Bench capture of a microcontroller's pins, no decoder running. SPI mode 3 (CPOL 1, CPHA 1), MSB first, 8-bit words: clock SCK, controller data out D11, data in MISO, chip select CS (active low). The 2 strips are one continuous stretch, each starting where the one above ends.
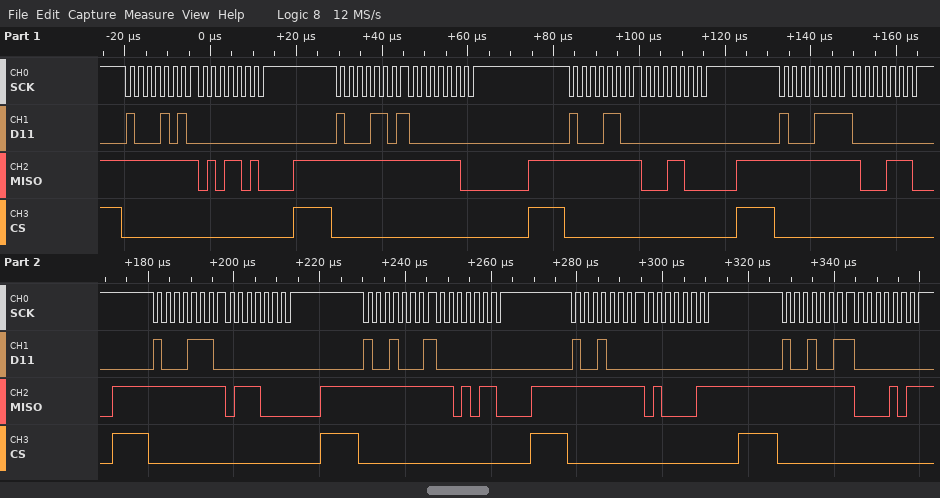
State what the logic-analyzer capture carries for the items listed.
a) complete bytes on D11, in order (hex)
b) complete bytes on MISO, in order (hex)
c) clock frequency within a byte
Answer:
8A 00 8D 00 8C 00 8F 00 8E 00 91 00 90 00 93 00
FF 5A FF FC FF 18 FF 8E FF 70 FF D6 FF 43 FF 0B
500 kHz
